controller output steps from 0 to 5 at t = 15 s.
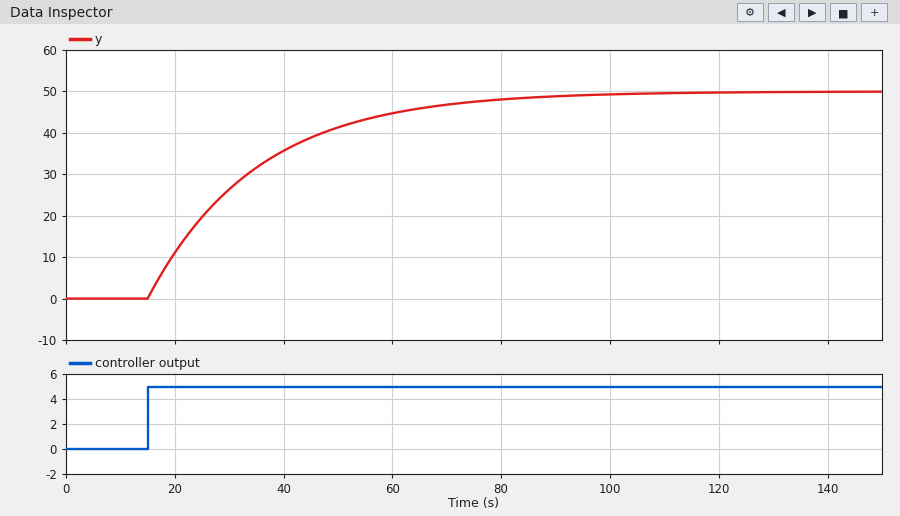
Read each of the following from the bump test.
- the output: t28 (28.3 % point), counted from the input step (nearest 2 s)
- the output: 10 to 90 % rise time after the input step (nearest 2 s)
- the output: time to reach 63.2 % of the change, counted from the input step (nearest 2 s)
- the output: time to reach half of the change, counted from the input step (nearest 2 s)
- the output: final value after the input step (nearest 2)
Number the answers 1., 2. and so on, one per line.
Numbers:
1. 6 s
2. 44 s
3. 20 s
4. 14 s
5. 50
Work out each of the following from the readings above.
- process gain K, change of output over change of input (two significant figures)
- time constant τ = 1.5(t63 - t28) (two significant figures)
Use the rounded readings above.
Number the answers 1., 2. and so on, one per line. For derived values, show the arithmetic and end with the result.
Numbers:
1. (50 - 0) / 5 = 10
2. 1.5 × (20 - 6) = 21 s
